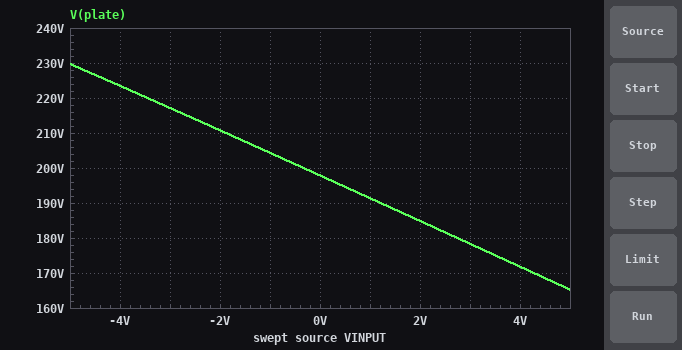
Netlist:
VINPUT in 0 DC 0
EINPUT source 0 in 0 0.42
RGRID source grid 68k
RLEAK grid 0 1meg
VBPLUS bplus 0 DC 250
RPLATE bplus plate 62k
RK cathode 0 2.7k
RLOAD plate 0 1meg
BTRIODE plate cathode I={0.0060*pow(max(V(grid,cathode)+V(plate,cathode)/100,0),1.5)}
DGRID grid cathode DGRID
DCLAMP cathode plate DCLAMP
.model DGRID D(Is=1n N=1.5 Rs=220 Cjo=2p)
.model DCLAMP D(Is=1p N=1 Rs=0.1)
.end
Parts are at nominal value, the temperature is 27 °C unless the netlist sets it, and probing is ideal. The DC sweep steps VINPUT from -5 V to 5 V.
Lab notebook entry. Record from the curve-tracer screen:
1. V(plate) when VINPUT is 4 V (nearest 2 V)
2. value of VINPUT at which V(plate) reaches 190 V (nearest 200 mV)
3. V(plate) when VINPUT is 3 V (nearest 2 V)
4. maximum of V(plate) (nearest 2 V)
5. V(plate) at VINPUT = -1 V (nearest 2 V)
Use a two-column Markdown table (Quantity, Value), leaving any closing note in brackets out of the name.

| Quantity | Value |
|---|---|
| V(plate) when VINPUT is 4 V | 172 V |
| value of VINPUT at which V(plate) reaches 190 V | 1.2 V |
| V(plate) when VINPUT is 3 V | 178 V |
| maximum of V(plate) | 230 V |
| V(plate) at VINPUT = -1 V | 204 V |
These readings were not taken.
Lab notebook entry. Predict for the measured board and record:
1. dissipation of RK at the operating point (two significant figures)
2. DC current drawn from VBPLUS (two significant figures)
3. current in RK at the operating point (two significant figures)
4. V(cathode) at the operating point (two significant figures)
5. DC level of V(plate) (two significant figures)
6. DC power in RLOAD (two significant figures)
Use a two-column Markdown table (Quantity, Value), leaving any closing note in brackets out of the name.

| Quantity | Value |
|---|---|
| dissipation of RK at the operating point | 1.1 mW |
| DC current drawn from VBPLUS | 840 µA |
| current in RK at the operating point | 640 µA |
| V(cathode) at the operating point | 1.7 V |
| DC level of V(plate) | 200 V |
| DC power in RLOAD | 39 mW |
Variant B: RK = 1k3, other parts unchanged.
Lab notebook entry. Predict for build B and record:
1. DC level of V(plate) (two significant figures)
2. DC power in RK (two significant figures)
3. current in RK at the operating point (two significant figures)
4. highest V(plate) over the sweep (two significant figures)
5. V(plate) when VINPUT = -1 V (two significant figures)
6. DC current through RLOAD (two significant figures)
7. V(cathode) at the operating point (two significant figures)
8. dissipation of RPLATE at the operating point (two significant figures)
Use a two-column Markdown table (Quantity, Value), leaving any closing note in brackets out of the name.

| Quantity | Value |
|---|---|
| DC level of V(plate) | 170 V |
| DC power in RK | 1.5 mW |
| current in RK at the operating point | 1.1 mA |
| highest V(plate) over the sweep | 230 V |
| V(plate) when VINPUT = -1 V | 180 V |
| DC current through RLOAD | 170 µA |
| V(cathode) at the operating point | 1.4 V |
| dissipation of RPLATE at the operating point | 96 mW |
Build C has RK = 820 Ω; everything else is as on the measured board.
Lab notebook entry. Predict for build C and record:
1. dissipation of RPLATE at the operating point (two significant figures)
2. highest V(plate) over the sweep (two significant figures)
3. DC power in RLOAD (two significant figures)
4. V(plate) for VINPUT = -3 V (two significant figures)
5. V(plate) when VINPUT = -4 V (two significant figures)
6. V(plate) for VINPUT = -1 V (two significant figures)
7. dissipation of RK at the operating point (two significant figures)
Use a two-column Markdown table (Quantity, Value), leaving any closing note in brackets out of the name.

| Quantity | Value |
|---|---|
| dissipation of RPLATE at the operating point | 150 mW |
| highest V(plate) over the sweep | 220 V |
| DC power in RLOAD | 24 mW |
| V(plate) for VINPUT = -3 V | 200 V |
| V(plate) when VINPUT = -4 V | 210 V |
| V(plate) for VINPUT = -1 V | 170 V |
| dissipation of RK at the operating point | 1.6 mW |
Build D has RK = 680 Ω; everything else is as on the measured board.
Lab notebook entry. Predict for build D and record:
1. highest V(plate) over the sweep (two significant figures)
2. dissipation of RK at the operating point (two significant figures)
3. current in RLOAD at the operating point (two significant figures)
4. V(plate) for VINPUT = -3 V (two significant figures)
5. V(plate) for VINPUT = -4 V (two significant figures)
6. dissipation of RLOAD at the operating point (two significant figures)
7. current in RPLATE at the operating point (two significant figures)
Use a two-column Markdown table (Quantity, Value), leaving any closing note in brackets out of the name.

| Quantity | Value |
|---|---|
| highest V(plate) over the sweep | 220 V |
| dissipation of RK at the operating point | 1.6 mW |
| current in RLOAD at the operating point | 150 µA |
| V(plate) for VINPUT = -3 V | 190 V |
| V(plate) for VINPUT = -4 V | 210 V |
| dissipation of RLOAD at the operating point | 21 mW |
| current in RPLATE at the operating point | 1.7 mA |
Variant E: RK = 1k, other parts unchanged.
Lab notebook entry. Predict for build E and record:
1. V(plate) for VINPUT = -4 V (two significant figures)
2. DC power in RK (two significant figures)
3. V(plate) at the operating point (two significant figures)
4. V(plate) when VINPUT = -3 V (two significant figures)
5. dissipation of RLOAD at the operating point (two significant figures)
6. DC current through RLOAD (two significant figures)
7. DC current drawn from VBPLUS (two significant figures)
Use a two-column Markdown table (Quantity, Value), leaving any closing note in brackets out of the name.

| Quantity | Value |
|---|---|
| V(plate) for VINPUT = -4 V | 210 V |
| DC power in RK | 1.6 mW |
| V(plate) at the operating point | 160 V |
| V(plate) when VINPUT = -3 V | 200 V |
| dissipation of RLOAD at the operating point | 26 mW |
| DC current through RLOAD | 160 µA |
| DC current drawn from VBPLUS | 1.4 mA |
